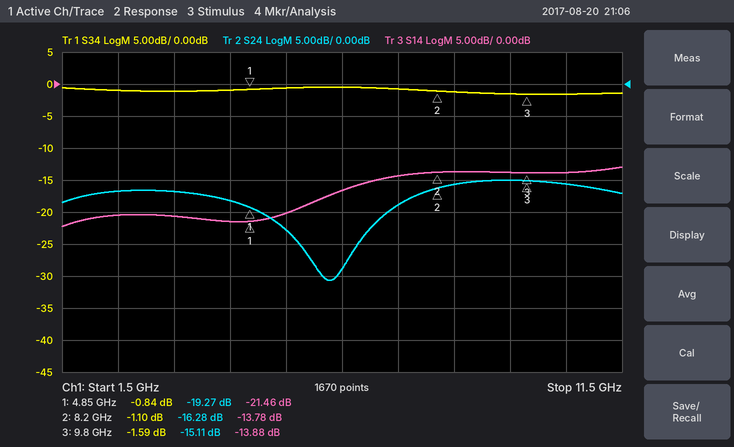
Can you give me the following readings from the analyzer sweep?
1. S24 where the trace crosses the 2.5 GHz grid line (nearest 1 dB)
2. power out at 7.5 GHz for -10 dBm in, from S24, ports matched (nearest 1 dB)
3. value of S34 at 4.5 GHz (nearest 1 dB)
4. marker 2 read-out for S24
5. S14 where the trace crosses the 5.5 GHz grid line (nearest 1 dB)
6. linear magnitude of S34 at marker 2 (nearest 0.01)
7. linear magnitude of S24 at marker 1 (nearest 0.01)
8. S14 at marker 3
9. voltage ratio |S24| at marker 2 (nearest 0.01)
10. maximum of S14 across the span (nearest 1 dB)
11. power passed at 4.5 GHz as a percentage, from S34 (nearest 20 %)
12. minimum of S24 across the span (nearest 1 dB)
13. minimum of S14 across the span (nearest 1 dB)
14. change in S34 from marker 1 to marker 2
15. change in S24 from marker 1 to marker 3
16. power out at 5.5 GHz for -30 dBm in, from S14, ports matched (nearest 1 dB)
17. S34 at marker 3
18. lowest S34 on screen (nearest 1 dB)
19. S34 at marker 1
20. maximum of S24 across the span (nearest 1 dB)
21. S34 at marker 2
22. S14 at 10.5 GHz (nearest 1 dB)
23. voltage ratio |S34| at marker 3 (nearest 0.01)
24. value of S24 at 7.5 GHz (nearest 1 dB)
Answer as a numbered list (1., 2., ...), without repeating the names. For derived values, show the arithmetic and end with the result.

1. -17 dB
2. -10 dBm + (-19 dB) = -29 dBm
3. -1 dB
4. -16.28 dB
5. -20 dB
6. 10^(-1.1/20) ≈ 0.88
7. 10^(-19.27/20) ≈ 0.11
8. -13.88 dB
9. 10^(-16.28/20) ≈ 0.15
10. -13 dB
11. 10^(-1/10) ≈ 79.4 %, so 80 % to the nearest 20 %
12. -31 dB
13. -22 dB
14. -1.1 − (-0.84) = -0.26 dB
15. -15.11 − (-19.27) = 4.16 dB
16. -30 dBm + (-20 dB) = -50 dBm
17. -1.59 dB
18. -2 dB
19. -0.84 dB
20. -15 dB
21. -1.10 dB
22. -14 dB
23. 10^(-1.59/20) ≈ 0.83
24. -19 dB
